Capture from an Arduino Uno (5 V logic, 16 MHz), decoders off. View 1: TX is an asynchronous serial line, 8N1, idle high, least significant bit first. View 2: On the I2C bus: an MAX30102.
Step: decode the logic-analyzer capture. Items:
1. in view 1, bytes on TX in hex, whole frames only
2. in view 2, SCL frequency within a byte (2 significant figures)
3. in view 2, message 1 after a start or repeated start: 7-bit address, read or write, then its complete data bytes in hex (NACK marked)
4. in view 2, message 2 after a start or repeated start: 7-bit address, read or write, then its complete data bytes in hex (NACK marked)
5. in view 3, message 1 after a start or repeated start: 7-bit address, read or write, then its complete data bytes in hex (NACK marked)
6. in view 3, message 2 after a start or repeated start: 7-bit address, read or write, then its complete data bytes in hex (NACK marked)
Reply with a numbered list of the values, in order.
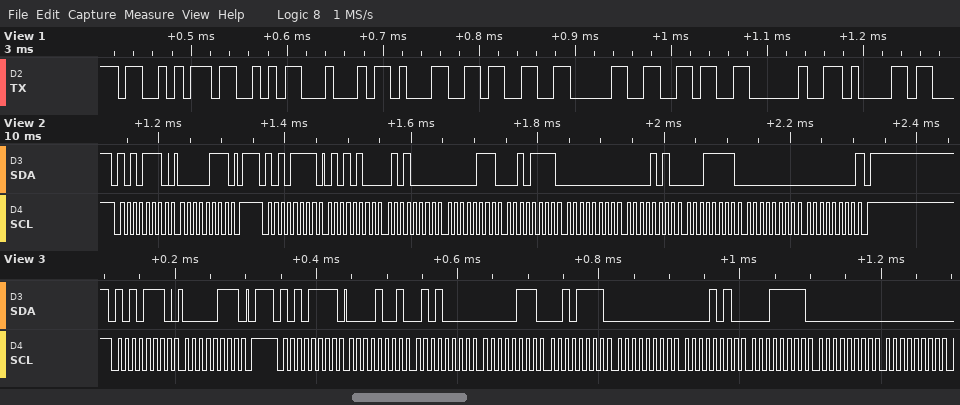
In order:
1. 53 53 44 31 33 30 36 20 61
2. 100 kHz
3. 0x57 write: 07
4. 0x57 read: 54 50 07 2F 00 0A 1F 00 00 NACK
5. 0x57 write: 07
6. 0x57 read: 09 50 07 2F 00 0A 1F 00 00
